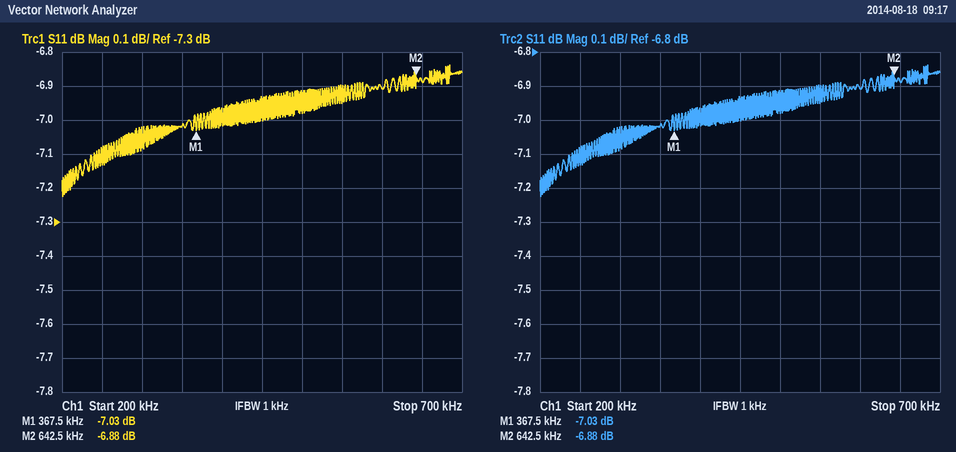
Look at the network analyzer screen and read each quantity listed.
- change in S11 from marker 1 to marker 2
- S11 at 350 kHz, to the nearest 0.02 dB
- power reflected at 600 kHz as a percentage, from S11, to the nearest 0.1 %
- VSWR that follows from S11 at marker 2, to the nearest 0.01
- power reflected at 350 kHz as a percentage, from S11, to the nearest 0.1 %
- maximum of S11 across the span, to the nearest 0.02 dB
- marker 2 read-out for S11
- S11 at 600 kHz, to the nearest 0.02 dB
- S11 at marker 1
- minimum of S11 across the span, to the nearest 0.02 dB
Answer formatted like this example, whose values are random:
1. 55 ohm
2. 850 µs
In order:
1. 0.15 dB
2. -7.02 dB
3. 20.4 %
4. 2.66
5. 19.9 %
6. -6.84 dB
7. -6.88 dB
8. -6.90 dB
9. -7.03 dB
10. -7.22 dB
